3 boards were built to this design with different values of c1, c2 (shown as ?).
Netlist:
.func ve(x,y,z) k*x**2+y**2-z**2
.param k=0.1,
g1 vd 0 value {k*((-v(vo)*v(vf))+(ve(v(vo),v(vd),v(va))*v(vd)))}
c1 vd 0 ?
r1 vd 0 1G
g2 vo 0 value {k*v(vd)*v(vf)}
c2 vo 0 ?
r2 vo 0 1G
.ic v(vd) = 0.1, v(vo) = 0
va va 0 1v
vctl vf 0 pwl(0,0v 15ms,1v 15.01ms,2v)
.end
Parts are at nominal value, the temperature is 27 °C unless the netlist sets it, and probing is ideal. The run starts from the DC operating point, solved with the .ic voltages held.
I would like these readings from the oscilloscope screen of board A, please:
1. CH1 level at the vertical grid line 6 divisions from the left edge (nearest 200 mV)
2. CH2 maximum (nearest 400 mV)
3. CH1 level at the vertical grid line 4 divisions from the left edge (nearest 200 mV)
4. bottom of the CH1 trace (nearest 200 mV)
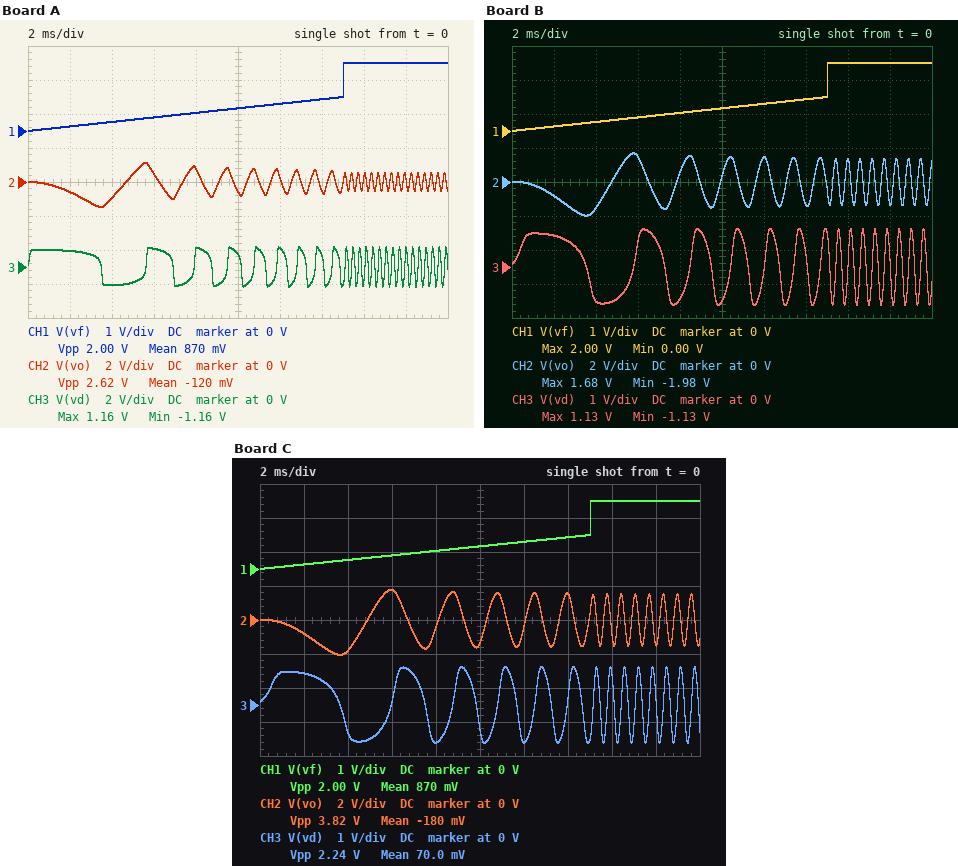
800 mV
1.2 V
600 mV
0 V
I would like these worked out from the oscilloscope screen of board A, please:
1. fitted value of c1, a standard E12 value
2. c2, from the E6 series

3.9 µF
22 µF
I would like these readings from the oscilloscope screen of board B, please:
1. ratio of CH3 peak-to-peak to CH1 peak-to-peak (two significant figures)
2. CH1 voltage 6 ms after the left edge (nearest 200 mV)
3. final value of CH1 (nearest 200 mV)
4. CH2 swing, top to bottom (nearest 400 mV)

1.1
400 mV
2.0 V
3.6 V
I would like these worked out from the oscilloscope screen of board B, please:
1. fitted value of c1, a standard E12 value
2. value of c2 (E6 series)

22 µF
15 µF
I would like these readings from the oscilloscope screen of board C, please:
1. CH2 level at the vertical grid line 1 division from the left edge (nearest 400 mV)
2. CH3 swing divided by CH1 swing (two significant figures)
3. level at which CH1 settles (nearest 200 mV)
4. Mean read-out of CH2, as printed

-800 mV
1.1
2.0 V
-180 mV
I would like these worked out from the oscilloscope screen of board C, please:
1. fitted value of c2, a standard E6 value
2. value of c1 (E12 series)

15 µF
27 µF
